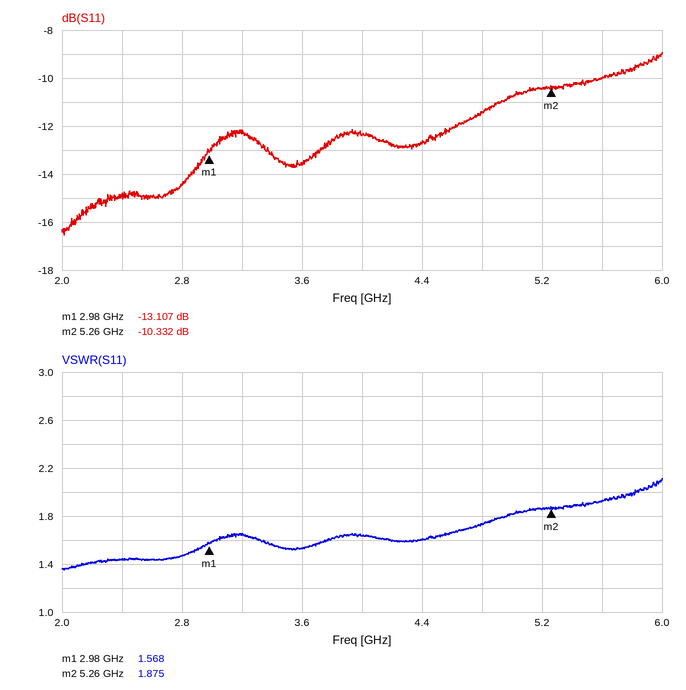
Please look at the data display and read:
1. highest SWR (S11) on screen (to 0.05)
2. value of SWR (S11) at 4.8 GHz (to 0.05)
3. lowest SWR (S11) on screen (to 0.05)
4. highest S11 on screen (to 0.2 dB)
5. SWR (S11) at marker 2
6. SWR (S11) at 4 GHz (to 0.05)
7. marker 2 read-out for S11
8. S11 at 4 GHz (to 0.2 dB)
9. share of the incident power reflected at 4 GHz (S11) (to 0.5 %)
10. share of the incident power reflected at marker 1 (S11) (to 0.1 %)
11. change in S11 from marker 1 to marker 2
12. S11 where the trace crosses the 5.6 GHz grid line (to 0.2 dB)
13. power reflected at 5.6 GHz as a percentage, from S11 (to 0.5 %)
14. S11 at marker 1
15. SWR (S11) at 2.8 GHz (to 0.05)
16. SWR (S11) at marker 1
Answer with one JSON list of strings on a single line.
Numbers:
["2.10", "1.75", "1.35", "-9.0 dB", "1.875", "1.65", "-10.332 dB", "-12.4 dB", "6.0 %", "4.9 %", "2.775 dB", "-10.0 dB", "10.0 %", "-13.107 dB", "1.45", "1.568"]
